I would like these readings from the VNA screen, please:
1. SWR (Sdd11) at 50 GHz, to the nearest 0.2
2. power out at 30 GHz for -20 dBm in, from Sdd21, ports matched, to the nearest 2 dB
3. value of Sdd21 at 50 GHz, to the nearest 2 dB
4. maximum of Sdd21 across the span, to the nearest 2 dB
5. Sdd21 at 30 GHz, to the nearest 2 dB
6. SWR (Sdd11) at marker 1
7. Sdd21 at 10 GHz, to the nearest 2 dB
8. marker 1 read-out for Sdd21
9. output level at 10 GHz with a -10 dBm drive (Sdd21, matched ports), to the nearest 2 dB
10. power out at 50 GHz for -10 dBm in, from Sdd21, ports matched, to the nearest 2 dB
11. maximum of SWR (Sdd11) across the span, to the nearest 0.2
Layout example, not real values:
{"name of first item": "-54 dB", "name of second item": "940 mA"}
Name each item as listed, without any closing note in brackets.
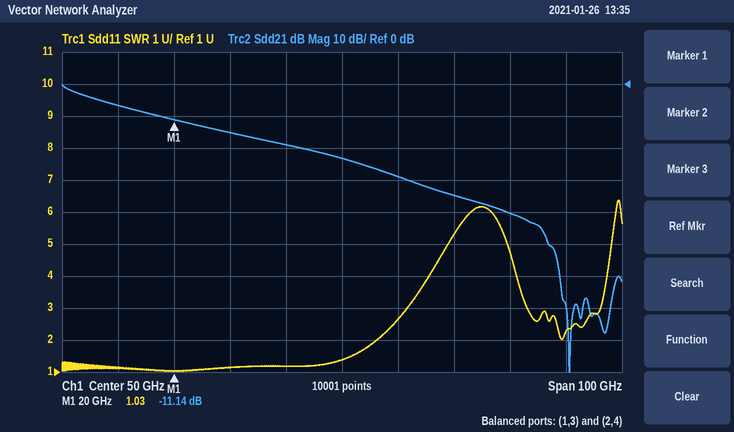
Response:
{"SWR (Sdd11) at 50 GHz, to the nearest 0.2": "1.4", "power out at 30 GHz for -20 dBm in, from Sdd21, ports matched, to the nearest 2 dB": "-36 dBm", "value of Sdd21 at 50 GHz, to the nearest 2 dB": "-24 dB", "maximum of Sdd21 across the span, to the nearest 2 dB": "0 dB", "Sdd21 at 30 GHz, to the nearest 2 dB": "-16 dB", "SWR (Sdd11) at marker 1": "1.03", "Sdd21 at 10 GHz, to the nearest 2 dB": "-6 dB", "marker 1 read-out for Sdd21": "-11.14 dB", "output level at 10 GHz with a -10 dBm drive (Sdd21, matched ports), to the nearest 2 dB": "-16 dBm", "power out at 50 GHz for -10 dBm in, from Sdd21, ports matched, to the nearest 2 dB": "-34 dBm", "maximum of SWR (Sdd11) across the span, to the nearest 0.2": "6.4"}
